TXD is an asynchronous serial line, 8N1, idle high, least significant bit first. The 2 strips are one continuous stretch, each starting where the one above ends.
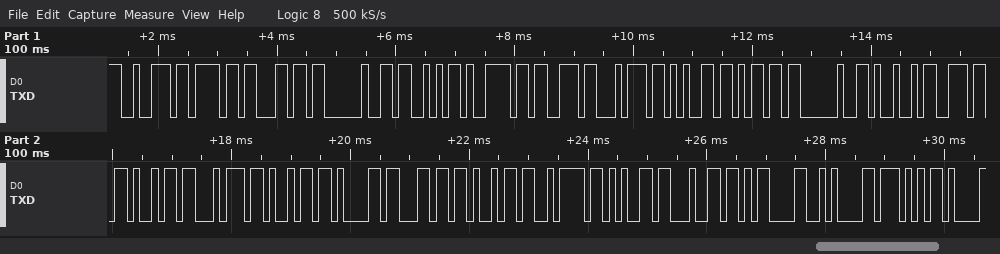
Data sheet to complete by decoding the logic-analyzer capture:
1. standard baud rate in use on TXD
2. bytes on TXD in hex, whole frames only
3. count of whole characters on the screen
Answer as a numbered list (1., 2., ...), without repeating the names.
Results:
1. 9600 baud
2. 72 6F 6C 20 53 79 73 74 65 6D 20 49 6E 69 74 69 61 6C 69 7A 65 64 0D 0A 57
3. 25
